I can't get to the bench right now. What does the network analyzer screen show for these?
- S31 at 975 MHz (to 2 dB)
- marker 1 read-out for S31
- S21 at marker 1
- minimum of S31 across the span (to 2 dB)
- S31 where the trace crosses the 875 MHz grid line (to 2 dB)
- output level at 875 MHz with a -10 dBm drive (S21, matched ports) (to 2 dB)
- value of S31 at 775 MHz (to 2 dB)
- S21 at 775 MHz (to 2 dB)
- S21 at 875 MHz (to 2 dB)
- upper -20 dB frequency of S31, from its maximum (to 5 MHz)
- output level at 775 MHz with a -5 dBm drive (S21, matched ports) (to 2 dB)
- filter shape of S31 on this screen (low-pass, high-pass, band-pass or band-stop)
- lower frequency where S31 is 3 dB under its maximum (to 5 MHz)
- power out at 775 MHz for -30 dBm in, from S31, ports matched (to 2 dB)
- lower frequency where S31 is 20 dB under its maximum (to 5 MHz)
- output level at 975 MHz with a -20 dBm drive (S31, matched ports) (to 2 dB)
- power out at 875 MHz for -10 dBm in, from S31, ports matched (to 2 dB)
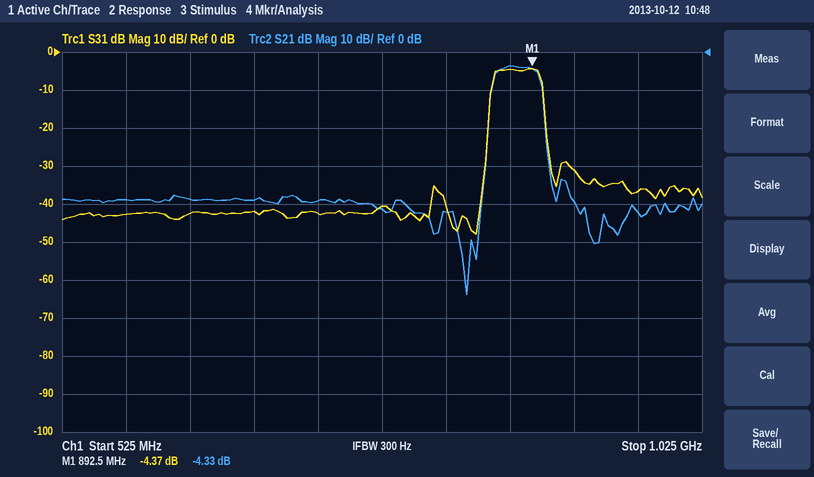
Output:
-36 dB
-4.37 dB
-4.33 dB
-48 dB
-4 dB
-14 dBm
-40 dB
-42 dB
-4 dB
905 MHz
-46 dBm
band-pass
860 MHz
-70 dBm
855 MHz
-56 dBm
-14 dBm
